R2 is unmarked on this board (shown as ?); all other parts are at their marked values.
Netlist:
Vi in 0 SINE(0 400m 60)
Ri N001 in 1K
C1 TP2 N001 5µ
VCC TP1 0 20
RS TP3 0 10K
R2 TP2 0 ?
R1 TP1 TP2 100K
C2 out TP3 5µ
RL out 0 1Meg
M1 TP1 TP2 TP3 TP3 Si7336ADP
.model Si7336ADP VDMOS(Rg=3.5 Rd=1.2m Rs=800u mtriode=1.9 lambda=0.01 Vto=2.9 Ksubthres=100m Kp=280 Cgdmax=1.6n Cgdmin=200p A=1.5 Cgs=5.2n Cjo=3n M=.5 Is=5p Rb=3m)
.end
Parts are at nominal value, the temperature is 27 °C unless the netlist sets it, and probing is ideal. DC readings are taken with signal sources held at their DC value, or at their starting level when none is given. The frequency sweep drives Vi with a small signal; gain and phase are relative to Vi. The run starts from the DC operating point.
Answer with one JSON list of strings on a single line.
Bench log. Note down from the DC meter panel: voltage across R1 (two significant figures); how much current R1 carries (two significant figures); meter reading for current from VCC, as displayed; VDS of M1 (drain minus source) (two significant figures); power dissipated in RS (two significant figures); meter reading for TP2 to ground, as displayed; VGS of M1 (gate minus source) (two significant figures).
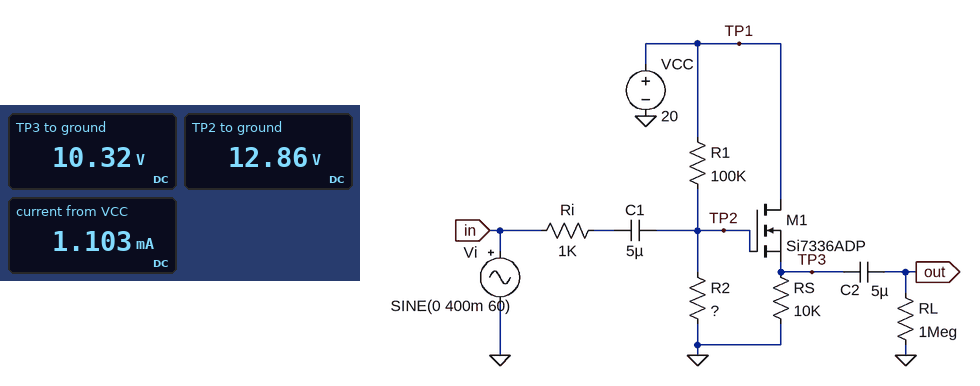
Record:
["7.1 V", "71 µA", "1.103 mA", "9.7 V", "11 mW", "12.86 V", "2.5 V"]
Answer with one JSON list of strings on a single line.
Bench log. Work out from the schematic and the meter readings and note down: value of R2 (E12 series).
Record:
["180 kΩ"]
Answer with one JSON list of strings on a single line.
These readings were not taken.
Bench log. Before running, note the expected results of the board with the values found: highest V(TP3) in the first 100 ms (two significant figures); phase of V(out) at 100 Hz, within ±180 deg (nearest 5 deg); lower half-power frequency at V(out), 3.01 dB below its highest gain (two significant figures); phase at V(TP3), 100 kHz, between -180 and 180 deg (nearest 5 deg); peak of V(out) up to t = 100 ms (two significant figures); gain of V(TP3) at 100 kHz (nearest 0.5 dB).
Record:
["11 V", "0 deg", "700 mHz", "-15 deg", "390 mV", "0.5 dB"]
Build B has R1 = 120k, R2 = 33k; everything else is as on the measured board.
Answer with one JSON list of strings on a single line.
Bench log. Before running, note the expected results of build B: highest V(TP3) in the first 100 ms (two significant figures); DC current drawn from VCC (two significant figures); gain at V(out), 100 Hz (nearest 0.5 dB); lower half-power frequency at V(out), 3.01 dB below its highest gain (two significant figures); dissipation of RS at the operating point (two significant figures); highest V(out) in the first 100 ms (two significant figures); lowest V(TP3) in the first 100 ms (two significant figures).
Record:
["2.2 V", "320 µA", "-0.5 dB", "1.3 Hz", "350 µW", "370 mV", "1.5 V"]
